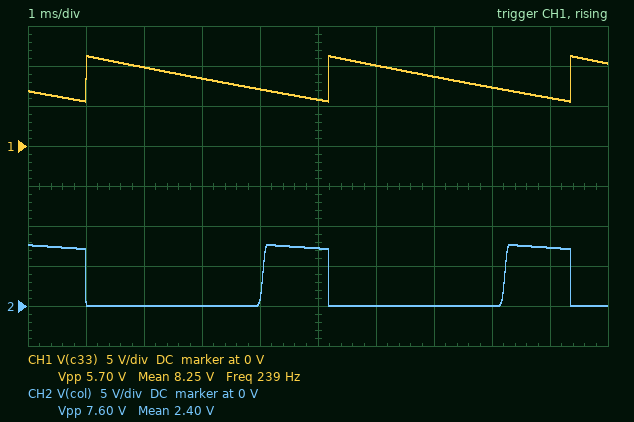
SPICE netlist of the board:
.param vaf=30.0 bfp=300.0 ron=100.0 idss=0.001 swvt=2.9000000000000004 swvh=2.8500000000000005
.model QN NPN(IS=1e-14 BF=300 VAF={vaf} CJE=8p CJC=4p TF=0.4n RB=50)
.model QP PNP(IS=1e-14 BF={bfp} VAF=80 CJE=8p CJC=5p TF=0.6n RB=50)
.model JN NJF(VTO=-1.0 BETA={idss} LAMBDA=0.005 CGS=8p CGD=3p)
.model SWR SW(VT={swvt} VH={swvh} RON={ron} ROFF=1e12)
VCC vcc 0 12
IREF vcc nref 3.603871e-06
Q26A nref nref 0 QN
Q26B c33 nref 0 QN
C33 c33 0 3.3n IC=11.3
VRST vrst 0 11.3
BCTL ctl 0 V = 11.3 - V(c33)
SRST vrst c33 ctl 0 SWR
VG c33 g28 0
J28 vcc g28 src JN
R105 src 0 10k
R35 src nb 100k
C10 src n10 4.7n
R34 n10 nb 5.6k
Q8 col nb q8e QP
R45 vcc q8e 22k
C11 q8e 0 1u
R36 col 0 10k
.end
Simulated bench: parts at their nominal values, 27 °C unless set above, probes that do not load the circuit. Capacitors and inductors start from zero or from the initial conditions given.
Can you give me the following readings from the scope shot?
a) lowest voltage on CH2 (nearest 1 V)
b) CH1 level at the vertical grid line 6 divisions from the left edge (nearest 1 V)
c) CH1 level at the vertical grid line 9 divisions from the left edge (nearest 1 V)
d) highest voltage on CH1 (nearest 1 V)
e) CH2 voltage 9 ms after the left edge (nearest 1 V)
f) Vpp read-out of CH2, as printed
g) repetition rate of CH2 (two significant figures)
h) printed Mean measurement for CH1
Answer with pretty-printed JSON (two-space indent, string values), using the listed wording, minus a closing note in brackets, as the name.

{
  "lowest voltage on CH2": "0 V",
  "CH1 level at the vertical grid line 6 divisions from the left edge": "10 V",
  "CH1 level at the vertical grid line 9 divisions from the left edge": "6 V",
  "highest voltage on CH1": "11 V",
  "CH2 voltage 9 ms after the left edge": "7 V",
  "Vpp read-out of CH2, as printed": "7.60 V",
  "repetition rate of CH2": "240 Hz",
  "printed Mean measurement for CH1": "8.25 V"
}
